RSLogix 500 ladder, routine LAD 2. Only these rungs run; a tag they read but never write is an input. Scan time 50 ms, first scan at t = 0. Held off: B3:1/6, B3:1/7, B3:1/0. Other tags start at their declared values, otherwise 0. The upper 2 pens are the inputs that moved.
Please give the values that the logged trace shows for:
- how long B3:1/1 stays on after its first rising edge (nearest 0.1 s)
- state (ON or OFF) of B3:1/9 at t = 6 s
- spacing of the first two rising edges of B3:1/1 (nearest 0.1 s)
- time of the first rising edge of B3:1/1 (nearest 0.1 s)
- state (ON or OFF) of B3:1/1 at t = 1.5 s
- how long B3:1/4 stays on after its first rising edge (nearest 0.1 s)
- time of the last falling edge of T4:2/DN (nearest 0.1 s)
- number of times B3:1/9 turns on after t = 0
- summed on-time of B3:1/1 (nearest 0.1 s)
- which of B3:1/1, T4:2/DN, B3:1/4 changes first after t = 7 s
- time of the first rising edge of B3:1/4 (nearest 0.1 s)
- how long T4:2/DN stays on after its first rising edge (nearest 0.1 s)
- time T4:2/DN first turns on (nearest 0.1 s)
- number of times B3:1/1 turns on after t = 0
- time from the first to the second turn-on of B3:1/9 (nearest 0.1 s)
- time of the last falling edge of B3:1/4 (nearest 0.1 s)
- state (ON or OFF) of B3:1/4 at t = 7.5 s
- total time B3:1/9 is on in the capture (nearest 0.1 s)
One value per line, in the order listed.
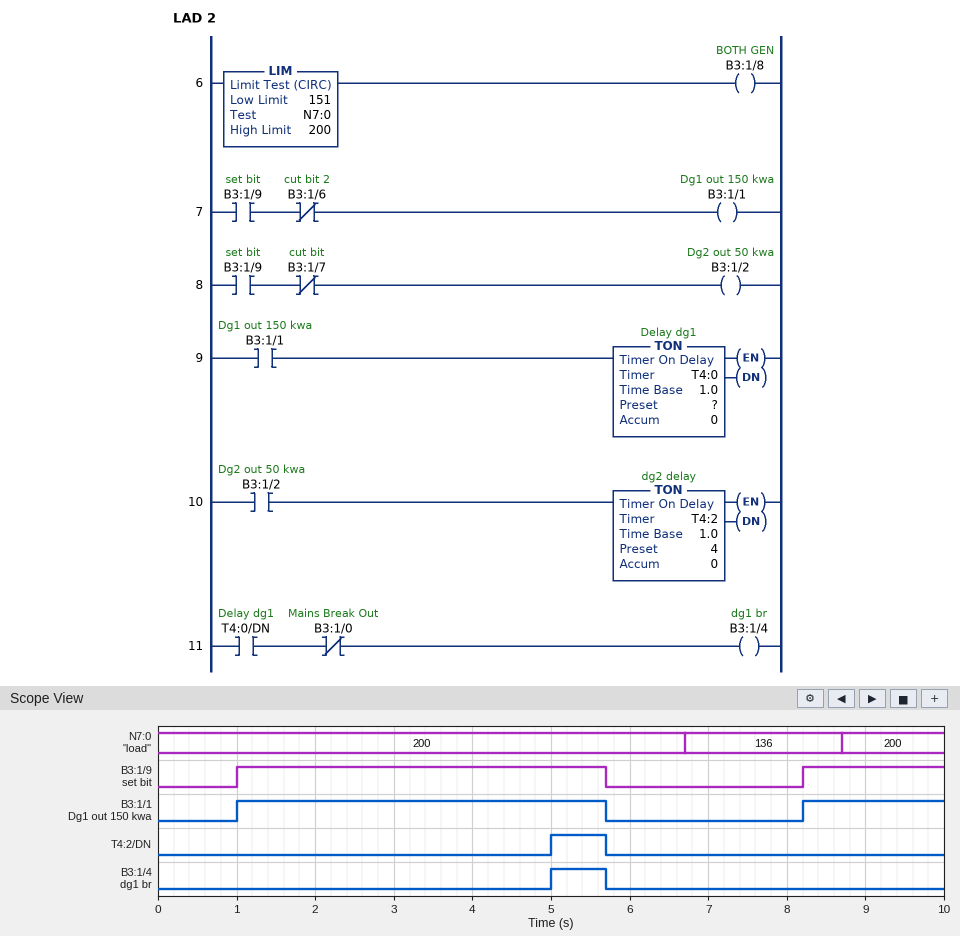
4.7 s
OFF
7.2 s
1.0 s
ON
0.7 s
5.7 s
2
6.5 s
B3:1/1
5.0 s
0.7 s
5.0 s
2
7.2 s
5.7 s
OFF
6.5 s
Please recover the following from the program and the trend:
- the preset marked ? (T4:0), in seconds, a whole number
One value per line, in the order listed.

4 s
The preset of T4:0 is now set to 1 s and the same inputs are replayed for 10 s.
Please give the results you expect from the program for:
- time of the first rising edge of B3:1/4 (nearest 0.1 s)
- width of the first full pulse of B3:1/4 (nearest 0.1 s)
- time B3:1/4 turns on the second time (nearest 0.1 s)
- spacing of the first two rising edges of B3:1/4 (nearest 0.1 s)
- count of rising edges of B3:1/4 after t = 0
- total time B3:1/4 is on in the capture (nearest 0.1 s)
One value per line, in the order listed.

2.0 s
3.7 s
9.2 s
7.2 s
2
4.5 s
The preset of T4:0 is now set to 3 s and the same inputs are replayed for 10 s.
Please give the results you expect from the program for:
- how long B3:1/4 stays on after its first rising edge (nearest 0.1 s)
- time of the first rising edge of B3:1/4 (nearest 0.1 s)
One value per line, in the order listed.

1.7 s
4.0 s
